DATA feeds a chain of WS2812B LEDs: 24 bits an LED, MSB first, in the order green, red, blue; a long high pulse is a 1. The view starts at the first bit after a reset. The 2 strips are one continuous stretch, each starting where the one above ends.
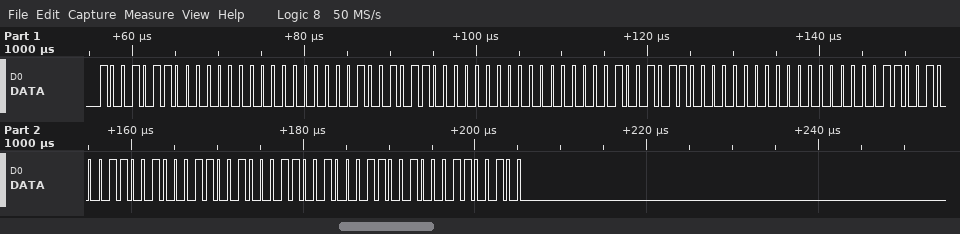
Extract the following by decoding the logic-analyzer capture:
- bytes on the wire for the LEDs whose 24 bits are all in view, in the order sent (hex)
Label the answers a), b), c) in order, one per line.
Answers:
a) 96 00 00 96 00 00 96 00 00 64 64 64 64 64 64
